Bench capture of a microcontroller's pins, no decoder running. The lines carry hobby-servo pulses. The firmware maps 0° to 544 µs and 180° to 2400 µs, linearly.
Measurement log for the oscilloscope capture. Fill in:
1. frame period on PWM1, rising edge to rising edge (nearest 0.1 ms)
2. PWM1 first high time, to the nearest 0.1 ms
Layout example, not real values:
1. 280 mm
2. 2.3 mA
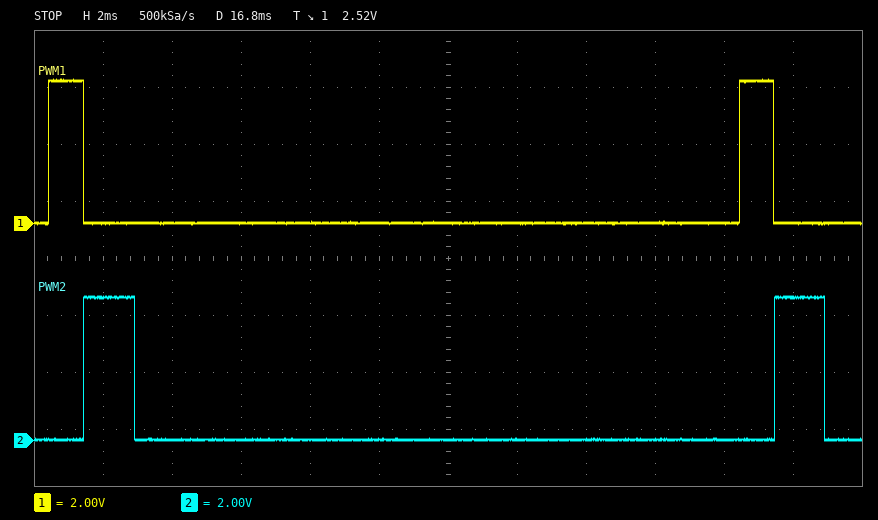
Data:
1. 20.0 ms
2. 1.0 ms
